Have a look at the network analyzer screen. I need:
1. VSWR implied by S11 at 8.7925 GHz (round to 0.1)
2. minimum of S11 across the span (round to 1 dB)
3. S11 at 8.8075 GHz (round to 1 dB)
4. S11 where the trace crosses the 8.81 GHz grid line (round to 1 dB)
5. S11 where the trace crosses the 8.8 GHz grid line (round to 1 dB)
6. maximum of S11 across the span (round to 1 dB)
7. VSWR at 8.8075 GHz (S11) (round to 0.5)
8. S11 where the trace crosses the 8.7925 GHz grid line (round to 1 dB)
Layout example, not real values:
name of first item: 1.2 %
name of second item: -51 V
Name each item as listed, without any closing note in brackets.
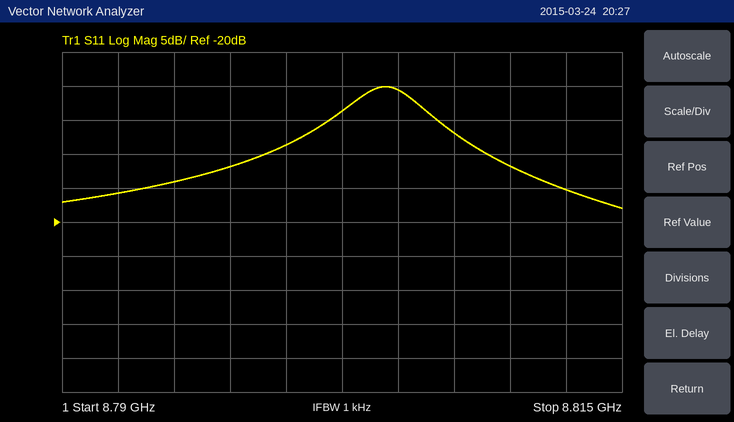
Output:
VSWR implied by S11 at 8.7925 GHz: 1.4
minimum of S11 across the span: -18 dB
S11 at 8.8075 GHz: -7 dB
S11 where the trace crosses the 8.81 GHz grid line: -12 dB
S11 where the trace crosses the 8.8 GHz grid line: -9 dB
maximum of S11 across the span: 0 dB
VSWR at 8.8075 GHz (S11): 2.5
S11 where the trace crosses the 8.7925 GHz grid line: -16 dB
